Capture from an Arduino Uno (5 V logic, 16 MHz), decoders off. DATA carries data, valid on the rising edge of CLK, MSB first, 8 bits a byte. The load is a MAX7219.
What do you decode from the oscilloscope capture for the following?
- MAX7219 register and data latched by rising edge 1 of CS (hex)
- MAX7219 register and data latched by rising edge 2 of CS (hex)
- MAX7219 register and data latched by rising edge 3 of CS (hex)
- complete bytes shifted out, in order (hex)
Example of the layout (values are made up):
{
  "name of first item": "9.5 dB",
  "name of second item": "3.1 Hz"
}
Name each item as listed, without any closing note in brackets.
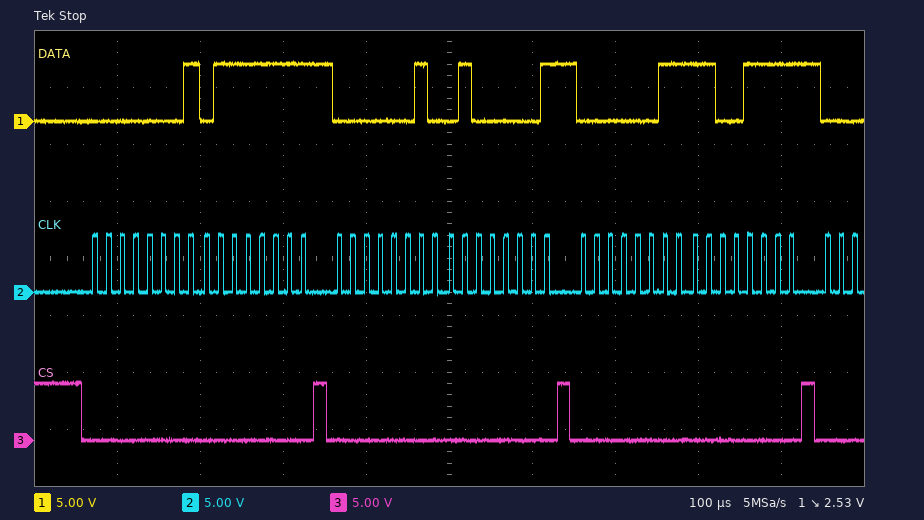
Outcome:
{
  "MAX7219 register and data latched by rising edge 1 of CS": "register 0x1, data 0x7F",
  "MAX7219 register and data latched by rising edge 2 of CS": "register 0x2, data 0x41",
  "MAX7219 register and data latched by rising edge 3 of CS": "register 0x3, data 0xCF",
  "complete bytes shifted out, in order": "01 7F 02 41 03 CF"
}
